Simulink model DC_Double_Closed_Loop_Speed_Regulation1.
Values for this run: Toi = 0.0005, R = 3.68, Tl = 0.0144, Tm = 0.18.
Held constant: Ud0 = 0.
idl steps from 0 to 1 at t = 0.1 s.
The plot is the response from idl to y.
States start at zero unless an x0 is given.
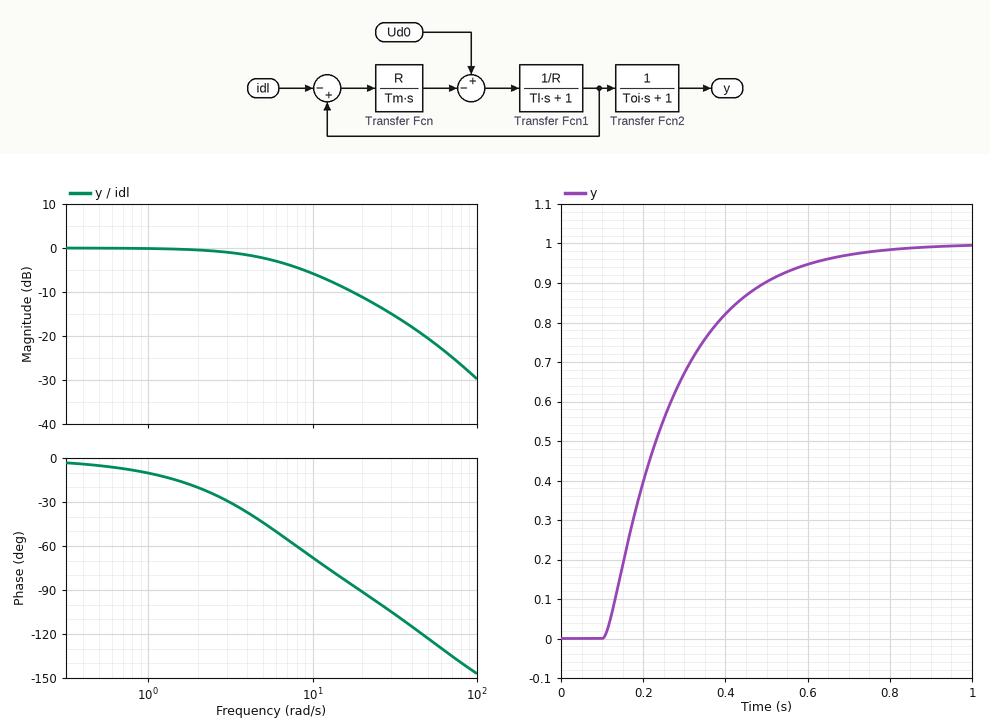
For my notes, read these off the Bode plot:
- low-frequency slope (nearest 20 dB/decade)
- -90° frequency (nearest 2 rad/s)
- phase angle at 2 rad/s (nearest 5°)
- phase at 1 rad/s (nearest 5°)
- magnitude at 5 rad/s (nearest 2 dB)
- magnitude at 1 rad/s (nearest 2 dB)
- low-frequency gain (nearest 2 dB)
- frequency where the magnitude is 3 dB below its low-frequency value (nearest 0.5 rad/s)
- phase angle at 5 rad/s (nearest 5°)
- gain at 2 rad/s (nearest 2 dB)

0 dB/decade
20 rad/s
-20°
-10°
-2 dB
0 dB
0 dB
6.0 rad/s
-45°
0 dB
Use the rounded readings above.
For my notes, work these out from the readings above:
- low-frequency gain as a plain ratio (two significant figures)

1.0
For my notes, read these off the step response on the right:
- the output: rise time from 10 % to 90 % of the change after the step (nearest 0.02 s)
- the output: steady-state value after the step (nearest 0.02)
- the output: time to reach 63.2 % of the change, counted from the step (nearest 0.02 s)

0.36 s
1.00
0.18 s
